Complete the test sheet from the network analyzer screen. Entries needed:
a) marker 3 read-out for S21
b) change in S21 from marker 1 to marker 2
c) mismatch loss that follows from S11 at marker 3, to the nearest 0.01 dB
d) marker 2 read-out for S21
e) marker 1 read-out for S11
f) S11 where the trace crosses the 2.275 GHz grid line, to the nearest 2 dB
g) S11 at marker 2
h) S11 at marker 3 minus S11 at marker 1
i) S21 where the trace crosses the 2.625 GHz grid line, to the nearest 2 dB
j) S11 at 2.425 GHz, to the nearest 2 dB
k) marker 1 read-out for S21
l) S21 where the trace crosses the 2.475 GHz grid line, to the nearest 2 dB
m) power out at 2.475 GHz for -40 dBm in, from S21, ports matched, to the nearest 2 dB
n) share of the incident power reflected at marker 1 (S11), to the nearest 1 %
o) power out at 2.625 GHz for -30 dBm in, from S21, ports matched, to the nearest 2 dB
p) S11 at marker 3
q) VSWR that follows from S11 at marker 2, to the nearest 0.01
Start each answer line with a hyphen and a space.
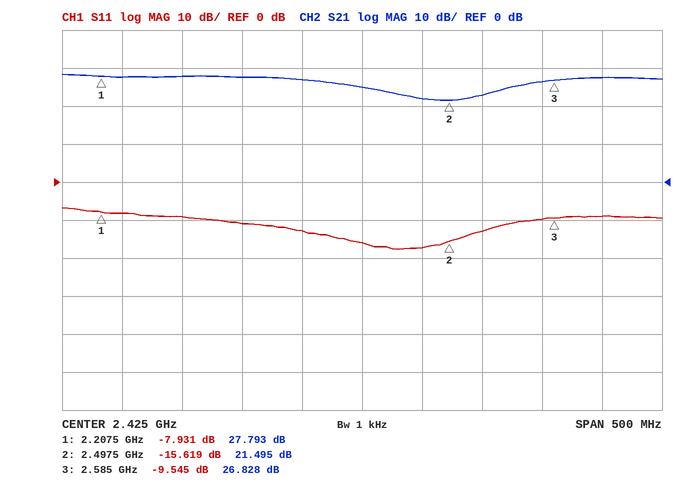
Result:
- 26.828 dB
- -6.298 dB
- 0.51 dB
- 21.495 dB
- -7.931 dB
- -10 dB
- -15.619 dB
- -1.614 dB
- 28 dB
- -16 dB
- 27.793 dB
- 22 dB
- -18 dBm
- 16 %
- -2 dBm
- -9.545 dB
- 1.40
